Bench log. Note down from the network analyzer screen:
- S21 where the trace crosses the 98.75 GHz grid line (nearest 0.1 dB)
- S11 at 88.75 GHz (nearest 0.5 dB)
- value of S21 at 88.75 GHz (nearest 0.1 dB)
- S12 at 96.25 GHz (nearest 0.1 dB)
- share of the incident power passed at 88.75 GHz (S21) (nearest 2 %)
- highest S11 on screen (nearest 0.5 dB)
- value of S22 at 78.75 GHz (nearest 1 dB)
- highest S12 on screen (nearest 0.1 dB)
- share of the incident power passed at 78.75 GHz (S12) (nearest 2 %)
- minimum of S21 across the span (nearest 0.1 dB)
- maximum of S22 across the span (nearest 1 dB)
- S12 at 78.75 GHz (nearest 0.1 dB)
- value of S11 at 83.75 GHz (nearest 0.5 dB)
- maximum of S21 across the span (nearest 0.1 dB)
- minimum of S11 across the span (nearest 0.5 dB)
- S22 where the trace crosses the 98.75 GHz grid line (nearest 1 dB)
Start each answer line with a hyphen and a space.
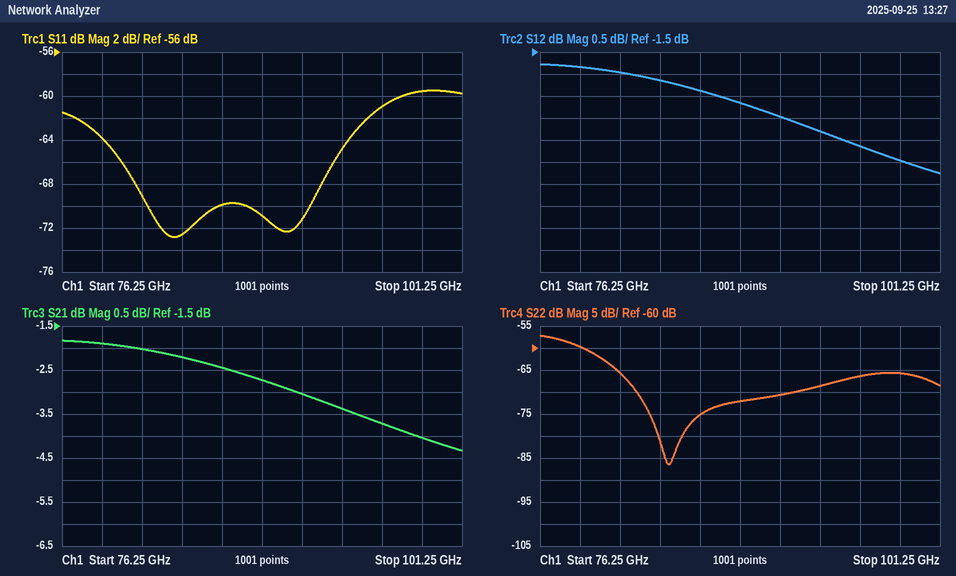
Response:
- -4.0 dB
- -71.0 dB
- -2.7 dB
- -3.6 dB
- 54 %
- -59.5 dB
- -60 dB
- -1.8 dB
- 66 %
- -4.3 dB
- -57 dB
- -1.8 dB
- -72.5 dB
- -1.8 dB
- -73.0 dB
- -66 dB
